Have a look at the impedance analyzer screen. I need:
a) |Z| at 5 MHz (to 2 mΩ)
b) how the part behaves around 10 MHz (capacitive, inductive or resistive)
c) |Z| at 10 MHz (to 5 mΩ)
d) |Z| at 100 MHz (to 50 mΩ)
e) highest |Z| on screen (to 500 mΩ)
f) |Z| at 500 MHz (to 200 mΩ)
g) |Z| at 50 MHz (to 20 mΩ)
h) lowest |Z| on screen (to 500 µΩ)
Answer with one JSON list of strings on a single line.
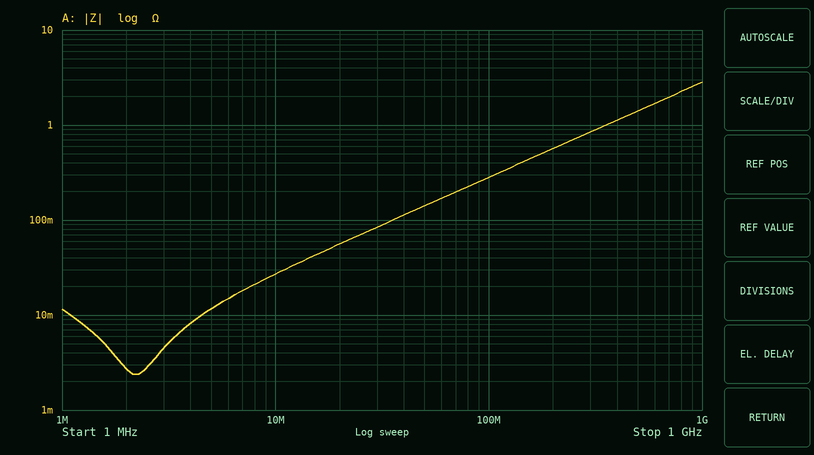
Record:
["12 mΩ", "inductive", "25 mΩ", "300 mΩ", "3.0 Ω", "1.4 Ω", "140 mΩ", "2.5 mΩ"]
